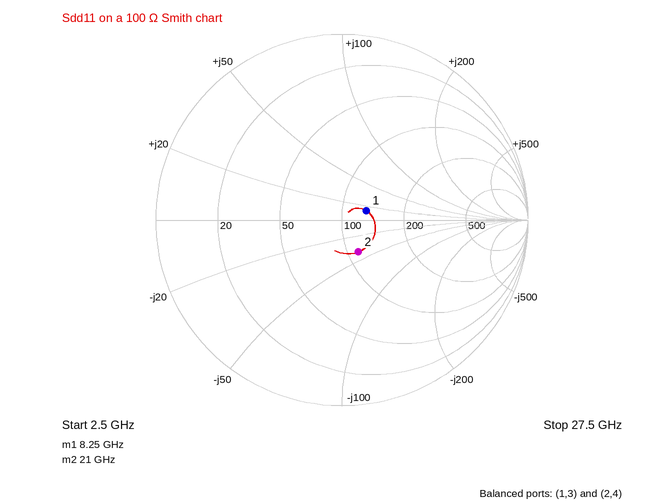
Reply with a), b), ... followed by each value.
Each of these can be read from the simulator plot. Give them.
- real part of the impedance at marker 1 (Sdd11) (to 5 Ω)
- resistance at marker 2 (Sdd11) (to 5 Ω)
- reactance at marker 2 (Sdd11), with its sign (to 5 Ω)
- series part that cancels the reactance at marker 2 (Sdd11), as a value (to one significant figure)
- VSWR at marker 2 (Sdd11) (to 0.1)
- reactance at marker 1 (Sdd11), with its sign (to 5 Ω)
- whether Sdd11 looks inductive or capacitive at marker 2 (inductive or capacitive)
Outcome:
a) 130 Ω
b) 110 Ω
c) -40 Ω
d) 300 pH
e) 1.5
f) +15 Ω
g) capacitive
